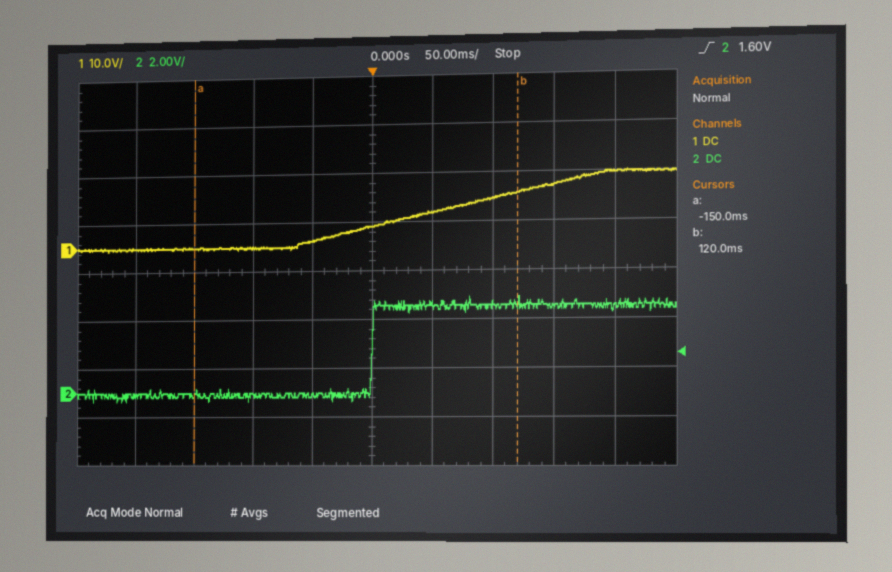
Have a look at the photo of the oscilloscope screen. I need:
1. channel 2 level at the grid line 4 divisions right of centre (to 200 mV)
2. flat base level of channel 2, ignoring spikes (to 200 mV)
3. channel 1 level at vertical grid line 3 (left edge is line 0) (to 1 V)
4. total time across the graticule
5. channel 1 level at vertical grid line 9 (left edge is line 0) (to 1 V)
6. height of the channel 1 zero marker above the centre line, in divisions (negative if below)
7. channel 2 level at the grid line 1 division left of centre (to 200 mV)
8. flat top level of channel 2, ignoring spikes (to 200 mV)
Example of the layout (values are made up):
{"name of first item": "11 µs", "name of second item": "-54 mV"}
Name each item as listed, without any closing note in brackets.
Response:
{"channel 2 level at the grid line 4 divisions right of centre": "3.4 V", "flat base level of channel 2, ignoring spikes": "0.0 V", "channel 1 level at vertical grid line 3 (left edge is line 0)": "0 V", "total time across the graticule": "500 ms", "channel 1 level at vertical grid line 9 (left edge is line 0)": "15 V", "height of the channel 1 zero marker above the centre line, in divisions": "+0.5 div", "channel 2 level at the grid line 1 division left of centre": "0.0 V", "flat top level of channel 2, ignoring spikes": "3.6 V"}
